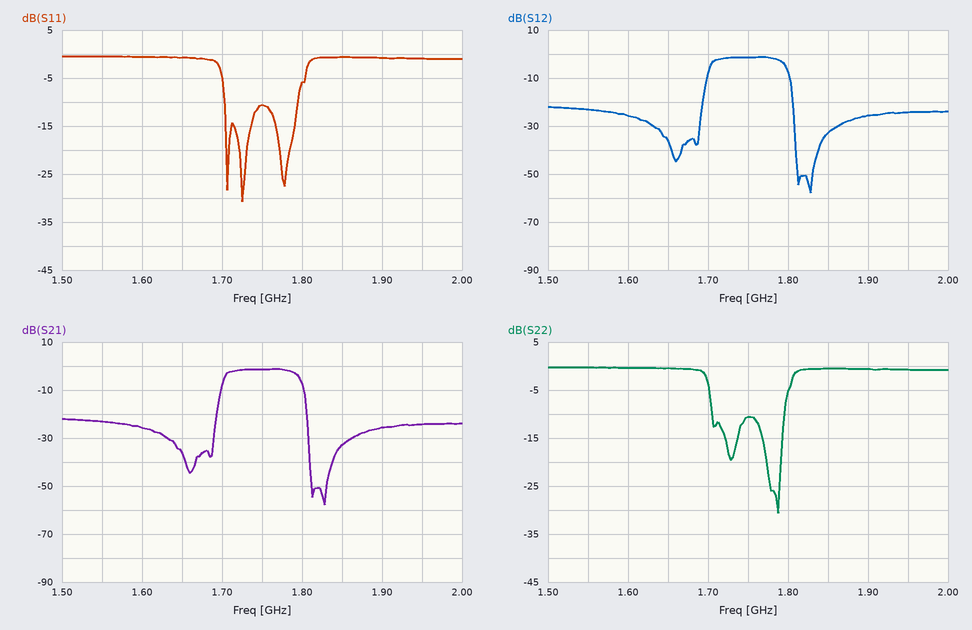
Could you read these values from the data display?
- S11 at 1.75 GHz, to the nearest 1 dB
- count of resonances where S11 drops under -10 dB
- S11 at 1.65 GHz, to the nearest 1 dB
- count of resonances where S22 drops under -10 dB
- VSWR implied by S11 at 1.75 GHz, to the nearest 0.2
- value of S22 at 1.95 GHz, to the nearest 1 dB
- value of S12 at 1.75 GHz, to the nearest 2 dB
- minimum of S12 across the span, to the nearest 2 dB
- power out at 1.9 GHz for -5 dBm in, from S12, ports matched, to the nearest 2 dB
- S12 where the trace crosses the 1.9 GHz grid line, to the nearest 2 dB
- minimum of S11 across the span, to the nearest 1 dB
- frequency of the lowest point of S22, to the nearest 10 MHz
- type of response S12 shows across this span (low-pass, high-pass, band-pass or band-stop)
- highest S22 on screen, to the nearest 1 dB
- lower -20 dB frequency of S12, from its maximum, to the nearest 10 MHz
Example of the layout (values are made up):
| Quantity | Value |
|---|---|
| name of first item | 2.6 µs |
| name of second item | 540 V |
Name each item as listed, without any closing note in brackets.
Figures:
| Quantity | Value |
|---|---|
| S11 at 1.75 GHz, to the nearest 1 dB | -11 dB |
| count of resonances where S11 drops under -10 dB | 3 |
| S11 at 1.65 GHz, to the nearest 1 dB | -1 dB |
| count of resonances where S22 drops under -10 dB | 2 |
| VSWR implied by S11 at 1.75 GHz, to the nearest 0.2 | 1.8 |
| value of S22 at 1.95 GHz, to the nearest 1 dB | -1 dB |
| value of S12 at 1.75 GHz, to the nearest 2 dB | -2 dB |
| minimum of S12 across the span, to the nearest 2 dB | -58 dB |
| power out at 1.9 GHz for -5 dBm in, from S12, ports matched, to the nearest 2 dB | -30 dBm |
| S12 where the trace crosses the 1.9 GHz grid line, to the nearest 2 dB | -26 dB |
| minimum of S11 across the span, to the nearest 1 dB | -31 dB |
| frequency of the lowest point of S22, to the nearest 10 MHz | 1.79 GHz |
| type of response S12 shows across this span | band-pass |
| highest S22 on screen, to the nearest 1 dB | 0 dB |
| lower -20 dB frequency of S12, from its maximum, to the nearest 10 MHz | 1.69 GHz |
